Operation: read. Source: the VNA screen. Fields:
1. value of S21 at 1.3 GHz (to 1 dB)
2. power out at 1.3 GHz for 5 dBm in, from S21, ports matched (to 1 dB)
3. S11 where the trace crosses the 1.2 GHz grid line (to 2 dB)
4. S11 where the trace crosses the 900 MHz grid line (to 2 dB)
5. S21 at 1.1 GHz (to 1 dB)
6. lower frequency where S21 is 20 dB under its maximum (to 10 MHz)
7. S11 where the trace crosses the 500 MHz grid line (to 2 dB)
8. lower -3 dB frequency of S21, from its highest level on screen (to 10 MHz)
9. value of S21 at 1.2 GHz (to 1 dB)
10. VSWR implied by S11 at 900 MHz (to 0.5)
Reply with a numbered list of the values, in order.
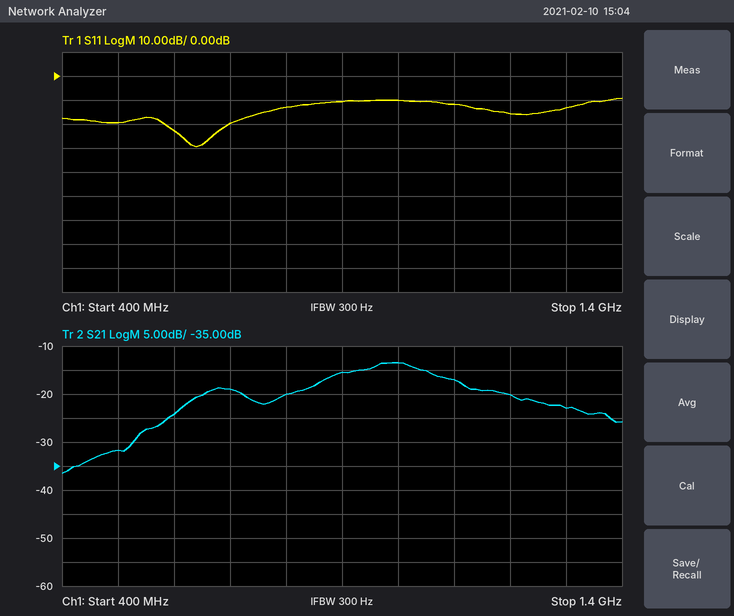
1. -23 dB
2. -18 dBm
3. -16 dB
4. -10 dB
5. -17 dB
6. 450 MHz
7. -20 dB
8. 880 MHz
9. -20 dB
10. 2.0
